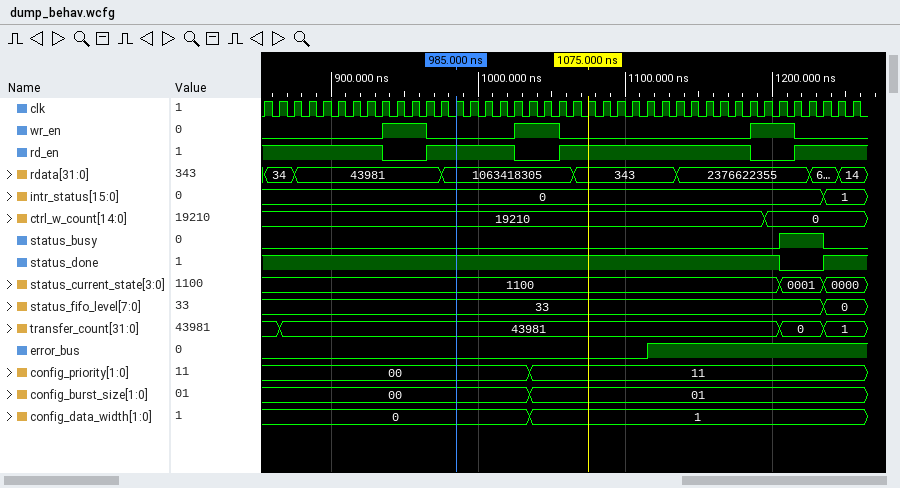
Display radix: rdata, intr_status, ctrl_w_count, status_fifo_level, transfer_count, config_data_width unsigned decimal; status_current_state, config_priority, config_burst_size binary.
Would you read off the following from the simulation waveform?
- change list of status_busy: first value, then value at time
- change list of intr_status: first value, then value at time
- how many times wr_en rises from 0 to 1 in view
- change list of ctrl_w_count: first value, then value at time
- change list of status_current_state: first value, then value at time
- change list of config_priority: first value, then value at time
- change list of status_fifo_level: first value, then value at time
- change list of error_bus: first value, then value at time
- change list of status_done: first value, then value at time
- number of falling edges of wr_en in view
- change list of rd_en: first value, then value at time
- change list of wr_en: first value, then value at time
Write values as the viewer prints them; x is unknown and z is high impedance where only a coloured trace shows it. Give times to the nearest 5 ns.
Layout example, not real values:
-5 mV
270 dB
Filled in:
0, 1 at 1205 ns, 0 at 1235 ns
0, 1 at 1235 ns
3
19210, 0 at 1195 ns
1100, 0001 at 1205 ns, 0000 at 1235 ns
00, 11 at 1035 ns
33, 0 at 1235 ns
0, 1 at 1115 ns
1, 0 at 1205 ns, 1 at 1235 ns
3
1, 0 at 935 ns, 1 at 965 ns, 0 at 1025 ns, 1 at 1055 ns, 0 at 1185 ns, 1 at 1215 ns
0, 1 at 935 ns, 0 at 965 ns, 1 at 1025 ns, 0 at 1055 ns, 1 at 1185 ns, 0 at 1215 ns
